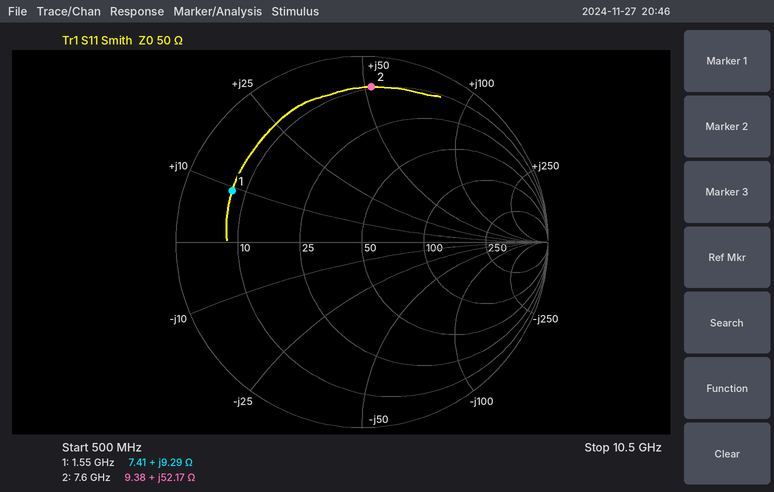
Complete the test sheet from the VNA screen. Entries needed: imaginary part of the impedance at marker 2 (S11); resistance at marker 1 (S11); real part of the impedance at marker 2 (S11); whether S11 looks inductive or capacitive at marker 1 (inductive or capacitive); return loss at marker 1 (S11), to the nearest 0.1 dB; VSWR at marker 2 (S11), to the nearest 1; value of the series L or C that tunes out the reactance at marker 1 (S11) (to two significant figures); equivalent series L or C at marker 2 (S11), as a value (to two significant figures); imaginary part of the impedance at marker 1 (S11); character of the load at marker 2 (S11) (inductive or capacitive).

+52.17 Ω
7.41 Ω
9.38 Ω
inductive
2.5 dB
11
11 pF
1.1 nH
+9.29 Ω
inductive
